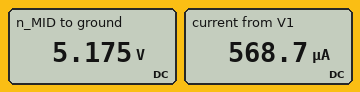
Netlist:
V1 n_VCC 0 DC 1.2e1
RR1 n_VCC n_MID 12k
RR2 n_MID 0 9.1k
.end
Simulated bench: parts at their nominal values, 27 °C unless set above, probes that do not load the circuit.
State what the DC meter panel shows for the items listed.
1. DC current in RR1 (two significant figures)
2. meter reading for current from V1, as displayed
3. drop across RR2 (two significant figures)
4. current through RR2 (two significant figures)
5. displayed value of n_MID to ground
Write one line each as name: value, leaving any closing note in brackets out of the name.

DC current in RR1: 570 µA
meter reading for current from V1, as displayed: 568.7 µA
drop across RR2: 5.2 V
current through RR2: 570 µA
displayed value of n_MID to ground: 5.175 V
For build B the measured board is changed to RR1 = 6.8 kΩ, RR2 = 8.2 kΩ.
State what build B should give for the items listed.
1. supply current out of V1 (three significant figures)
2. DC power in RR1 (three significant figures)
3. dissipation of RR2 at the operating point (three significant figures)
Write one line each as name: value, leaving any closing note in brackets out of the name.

supply current out of V1: 800 µA
DC power in RR1: 4.35 mW
dissipation of RR2 at the operating point: 5.25 mW
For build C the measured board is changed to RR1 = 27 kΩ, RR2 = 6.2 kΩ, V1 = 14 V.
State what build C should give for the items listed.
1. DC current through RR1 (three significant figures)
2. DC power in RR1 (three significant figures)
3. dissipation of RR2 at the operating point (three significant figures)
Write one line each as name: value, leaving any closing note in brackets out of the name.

DC current through RR1: 422 µA
DC power in RR1: 4.80 mW
dissipation of RR2 at the operating point: 1.10 mW
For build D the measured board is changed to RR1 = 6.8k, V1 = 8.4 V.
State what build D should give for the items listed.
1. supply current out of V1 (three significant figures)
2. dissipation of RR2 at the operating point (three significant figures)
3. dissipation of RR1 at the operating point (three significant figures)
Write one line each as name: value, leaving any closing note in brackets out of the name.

supply current out of V1: 528 µA
dissipation of RR2 at the operating point: 2.54 mW
dissipation of RR1 at the operating point: 1.90 mW
